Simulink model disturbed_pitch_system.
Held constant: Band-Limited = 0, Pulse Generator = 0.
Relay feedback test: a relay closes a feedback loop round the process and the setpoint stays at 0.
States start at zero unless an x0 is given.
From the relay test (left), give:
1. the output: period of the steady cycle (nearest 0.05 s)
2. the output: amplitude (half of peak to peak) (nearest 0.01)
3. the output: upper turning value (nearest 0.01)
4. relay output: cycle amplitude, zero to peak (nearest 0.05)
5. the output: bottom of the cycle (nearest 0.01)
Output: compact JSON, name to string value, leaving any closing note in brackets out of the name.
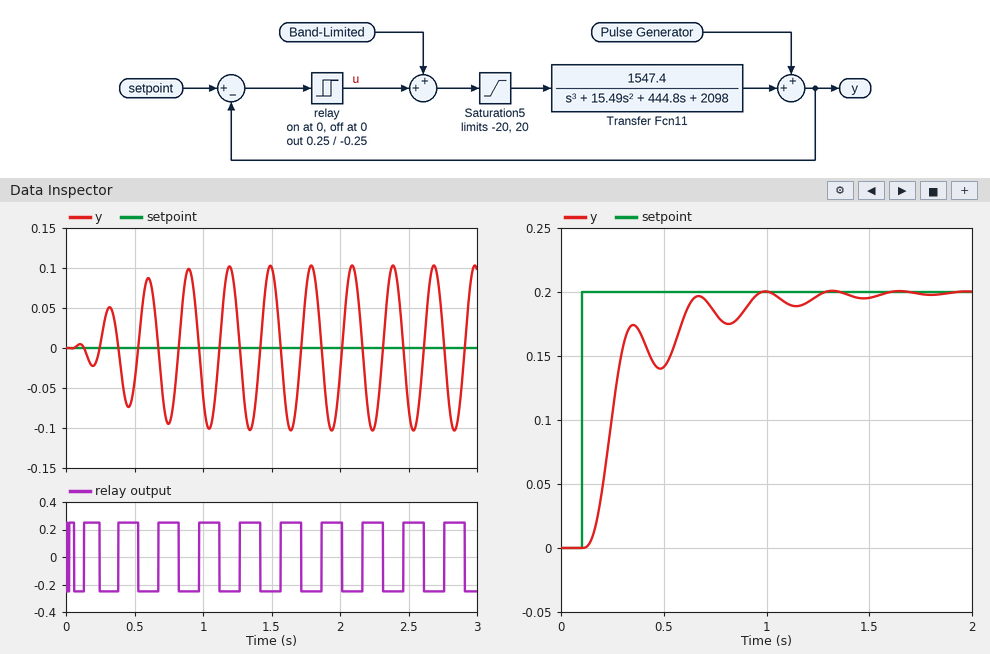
{"the output: period of the steady cycle": "0.30 s", "the output: amplitude (half of peak to peak)": "0.10", "the output: upper turning value": "0.10", "relay output: cycle amplitude, zero to peak": "0.25", "the output: bottom of the cycle": "-0.10"}
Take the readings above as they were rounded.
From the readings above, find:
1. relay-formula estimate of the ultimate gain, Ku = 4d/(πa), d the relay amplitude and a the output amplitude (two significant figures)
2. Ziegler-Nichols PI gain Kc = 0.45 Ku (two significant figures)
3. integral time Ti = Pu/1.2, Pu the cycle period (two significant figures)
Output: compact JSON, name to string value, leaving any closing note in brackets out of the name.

{"relay-formula estimate of the ultimate gain, Ku = 4d/(πa), d the relay amplitude and a the output amplitude": "3.2", "Ziegler-Nichols PI gain Kc = 0.45 Ku": "1.4", "integral time Ti = Pu/1.2, Pu the cycle period": "0.25 s"}
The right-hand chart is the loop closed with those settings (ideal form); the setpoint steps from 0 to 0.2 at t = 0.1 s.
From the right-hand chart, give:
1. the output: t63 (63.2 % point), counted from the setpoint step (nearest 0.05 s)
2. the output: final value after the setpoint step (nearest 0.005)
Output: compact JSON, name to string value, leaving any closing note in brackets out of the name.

{"the output: t63 (63.2 % point), counted from the setpoint step": "0.15 s", "the output: final value after the setpoint step": "0.200"}
